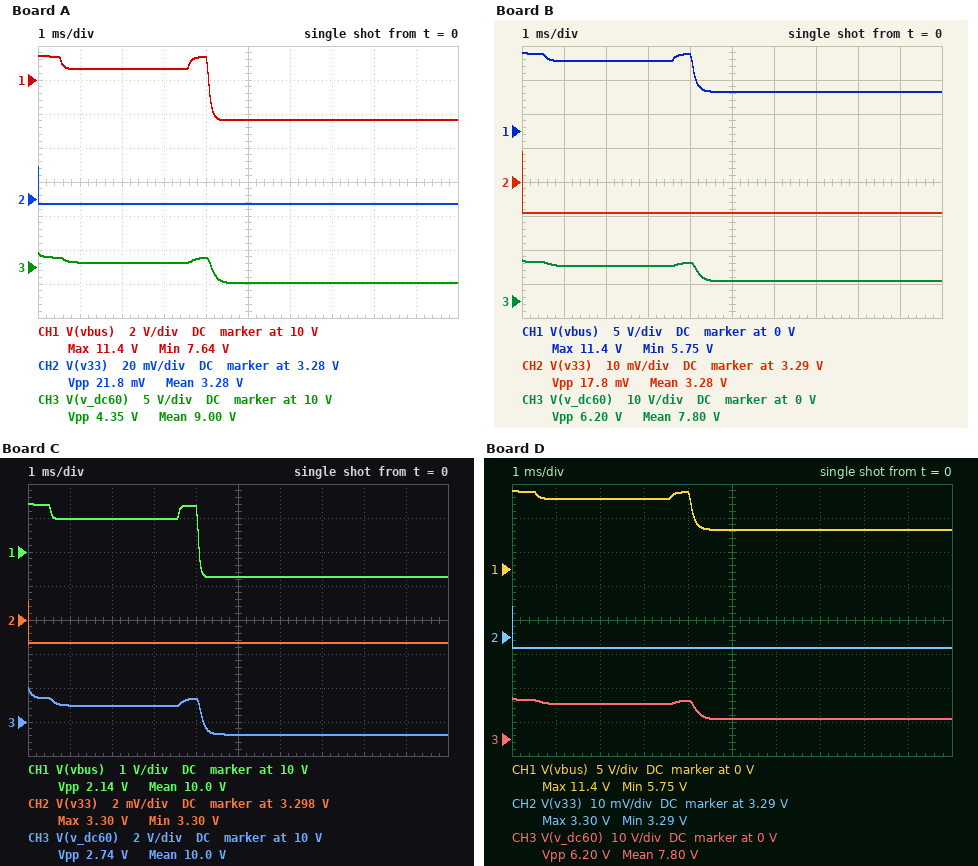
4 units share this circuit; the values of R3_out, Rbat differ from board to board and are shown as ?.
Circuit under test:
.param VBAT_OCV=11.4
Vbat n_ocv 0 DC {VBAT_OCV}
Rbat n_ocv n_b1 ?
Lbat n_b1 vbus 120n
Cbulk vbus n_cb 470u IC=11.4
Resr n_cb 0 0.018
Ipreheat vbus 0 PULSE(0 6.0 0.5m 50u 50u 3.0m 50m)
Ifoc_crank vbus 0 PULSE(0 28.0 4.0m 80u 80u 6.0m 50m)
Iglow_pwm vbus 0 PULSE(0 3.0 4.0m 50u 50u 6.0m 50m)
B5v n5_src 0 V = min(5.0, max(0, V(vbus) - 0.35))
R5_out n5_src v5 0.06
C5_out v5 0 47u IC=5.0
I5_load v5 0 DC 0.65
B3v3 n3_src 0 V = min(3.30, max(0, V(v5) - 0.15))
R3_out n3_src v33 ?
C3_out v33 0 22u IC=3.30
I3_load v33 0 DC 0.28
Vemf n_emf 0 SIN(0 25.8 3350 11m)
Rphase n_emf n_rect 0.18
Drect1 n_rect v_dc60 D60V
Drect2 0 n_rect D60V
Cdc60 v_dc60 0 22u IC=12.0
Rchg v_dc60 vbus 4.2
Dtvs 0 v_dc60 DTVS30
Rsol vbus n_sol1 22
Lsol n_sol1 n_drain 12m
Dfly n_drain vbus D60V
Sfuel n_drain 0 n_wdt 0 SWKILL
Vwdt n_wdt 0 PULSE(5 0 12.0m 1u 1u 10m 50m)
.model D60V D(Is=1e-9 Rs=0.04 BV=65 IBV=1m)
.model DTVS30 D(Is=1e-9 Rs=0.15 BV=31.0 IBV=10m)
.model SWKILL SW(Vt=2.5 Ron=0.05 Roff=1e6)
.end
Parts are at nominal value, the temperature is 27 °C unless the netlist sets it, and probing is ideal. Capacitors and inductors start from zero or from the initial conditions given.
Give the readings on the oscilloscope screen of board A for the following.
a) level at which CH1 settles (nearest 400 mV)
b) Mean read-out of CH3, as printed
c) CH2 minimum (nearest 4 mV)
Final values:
7.6 V
9.00 V
3.276 V
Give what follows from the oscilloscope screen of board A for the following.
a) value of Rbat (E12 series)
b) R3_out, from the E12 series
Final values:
0.12 Ω
0.082 Ω
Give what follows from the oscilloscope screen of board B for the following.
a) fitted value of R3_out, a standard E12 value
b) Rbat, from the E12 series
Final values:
0.068 Ω
0.18 Ω
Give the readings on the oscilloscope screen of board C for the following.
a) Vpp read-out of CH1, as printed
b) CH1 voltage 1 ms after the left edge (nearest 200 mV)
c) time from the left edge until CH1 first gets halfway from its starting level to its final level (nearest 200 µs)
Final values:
2.14 V
11.0 V
4.0 ms
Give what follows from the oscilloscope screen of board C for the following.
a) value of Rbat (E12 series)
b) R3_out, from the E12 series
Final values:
0.068 Ω
0.012 Ω
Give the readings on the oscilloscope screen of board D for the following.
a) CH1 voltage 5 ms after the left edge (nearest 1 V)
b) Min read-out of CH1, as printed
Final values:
6 V
5.75 V
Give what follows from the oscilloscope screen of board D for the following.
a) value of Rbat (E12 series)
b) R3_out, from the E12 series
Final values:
0.18 Ω
0.047 Ω
